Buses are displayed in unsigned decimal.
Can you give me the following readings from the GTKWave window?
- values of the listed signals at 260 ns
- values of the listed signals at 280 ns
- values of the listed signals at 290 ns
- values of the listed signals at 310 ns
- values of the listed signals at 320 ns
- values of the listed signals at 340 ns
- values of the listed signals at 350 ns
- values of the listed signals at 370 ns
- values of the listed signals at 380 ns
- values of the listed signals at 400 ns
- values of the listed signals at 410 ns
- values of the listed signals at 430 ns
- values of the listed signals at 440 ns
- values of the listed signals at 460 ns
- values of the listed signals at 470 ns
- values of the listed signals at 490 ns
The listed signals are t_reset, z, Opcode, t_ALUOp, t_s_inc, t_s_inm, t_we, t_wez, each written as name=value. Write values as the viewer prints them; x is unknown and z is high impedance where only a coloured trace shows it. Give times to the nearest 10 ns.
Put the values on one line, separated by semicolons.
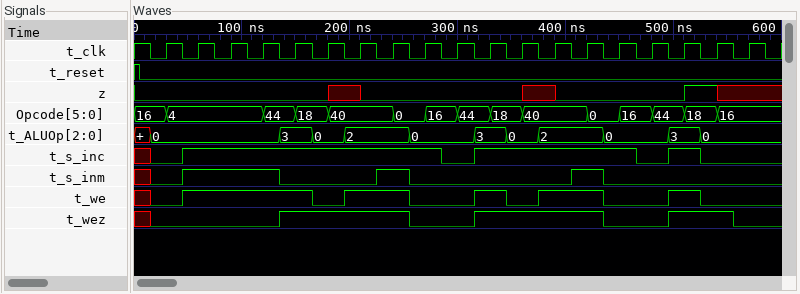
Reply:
t_reset=0, z=0, Opcode=0, t_ALUOp=0, t_s_inc=1, t_s_inm=0, t_we=0, t_wez=0; t_reset=0, z=0, Opcode=16, t_ALUOp=0, t_s_inc=1, t_s_inm=0, t_we=0, t_wez=0; t_reset=0, z=0, Opcode=16, t_ALUOp=0, t_s_inc=0, t_s_inm=0, t_we=0, t_wez=0; t_reset=0, z=0, Opcode=44, t_ALUOp=0, t_s_inc=0, t_s_inm=0, t_we=0, t_wez=0; t_reset=0, z=0, Opcode=44, t_ALUOp=3, t_s_inc=1, t_s_inm=0, t_we=1, t_wez=1; t_reset=0, z=0, Opcode=18, t_ALUOp=3, t_s_inc=1, t_s_inm=0, t_we=1, t_wez=1; t_reset=0, z=0, Opcode=18, t_ALUOp=0, t_s_inc=1, t_s_inm=0, t_we=0, t_wez=1; t_reset=0, z=x, Opcode=40, t_ALUOp=0, t_s_inc=1, t_s_inm=0, t_we=0, t_wez=1; t_reset=0, z=x, Opcode=40, t_ALUOp=2, t_s_inc=1, t_s_inm=0, t_we=1, t_wez=1; t_reset=0, z=0, Opcode=40, t_ALUOp=2, t_s_inc=1, t_s_inm=0, t_we=1, t_wez=1; t_reset=0, z=0, Opcode=40, t_ALUOp=2, t_s_inc=1, t_s_inm=1, t_we=1, t_wez=1; t_reset=0, z=0, Opcode=0, t_ALUOp=2, t_s_inc=1, t_s_inm=1, t_we=1, t_wez=1; t_reset=0, z=0, Opcode=0, t_ALUOp=0, t_s_inc=1, t_s_inm=0, t_we=0, t_wez=0; t_reset=0, z=0, Opcode=16, t_ALUOp=0, t_s_inc=1, t_s_inm=0, t_we=0, t_wez=0; t_reset=0, z=0, Opcode=16, t_ALUOp=0, t_s_inc=0, t_s_inm=0, t_we=0, t_wez=0; t_reset=0, z=0, Opcode=44, t_ALUOp=0, t_s_inc=0, t_s_inm=0, t_we=0, t_wez=0
